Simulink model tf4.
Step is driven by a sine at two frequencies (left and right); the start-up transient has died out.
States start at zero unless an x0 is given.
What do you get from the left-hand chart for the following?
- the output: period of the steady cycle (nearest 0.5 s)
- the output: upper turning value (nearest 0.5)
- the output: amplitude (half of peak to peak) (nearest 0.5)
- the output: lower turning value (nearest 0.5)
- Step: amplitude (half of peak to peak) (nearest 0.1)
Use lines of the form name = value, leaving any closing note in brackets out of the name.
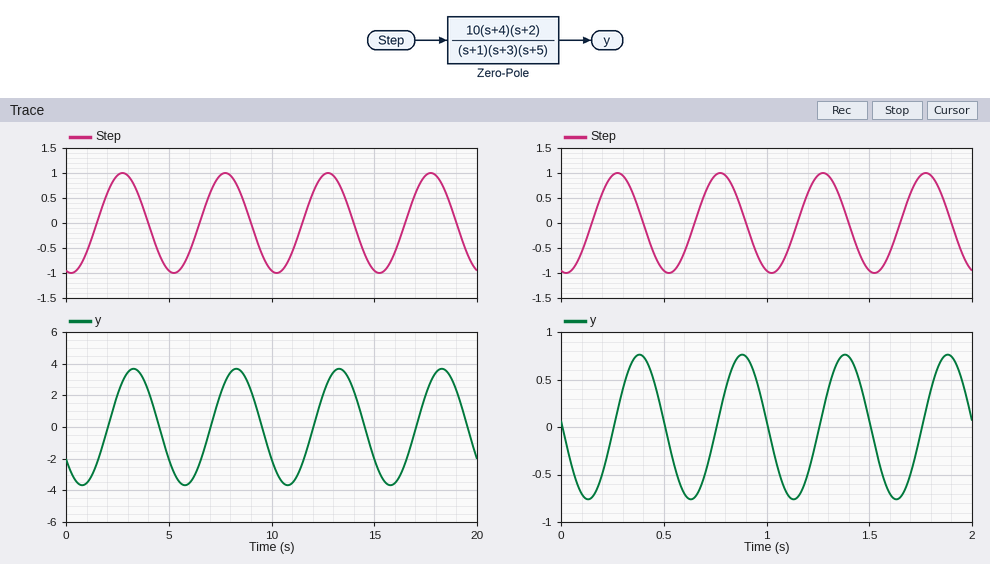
the output: period of the steady cycle = 5.0 s
the output: upper turning value = 3.5
the output: amplitude (half of peak to peak) = 3.5
the output: lower turning value = -3.5
Step: amplitude (half of peak to peak) = 1.0
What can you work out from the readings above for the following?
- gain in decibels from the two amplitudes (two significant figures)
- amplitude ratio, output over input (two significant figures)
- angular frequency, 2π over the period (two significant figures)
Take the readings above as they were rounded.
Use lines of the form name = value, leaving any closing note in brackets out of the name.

gain in decibels from the two amplitudes = 11 dB
amplitude ratio, output over input = 3.5
angular frequency, 2π over the period = 1.3 rad/s
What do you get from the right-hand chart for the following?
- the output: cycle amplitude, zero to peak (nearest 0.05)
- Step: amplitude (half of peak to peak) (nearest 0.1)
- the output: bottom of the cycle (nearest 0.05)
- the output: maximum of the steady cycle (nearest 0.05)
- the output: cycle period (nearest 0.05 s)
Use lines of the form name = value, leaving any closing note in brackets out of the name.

the output: cycle amplitude, zero to peak = 0.75
Step: amplitude (half of peak to peak) = 1.0
the output: bottom of the cycle = -0.75
the output: maximum of the steady cycle = 0.75
the output: cycle period = 0.50 s
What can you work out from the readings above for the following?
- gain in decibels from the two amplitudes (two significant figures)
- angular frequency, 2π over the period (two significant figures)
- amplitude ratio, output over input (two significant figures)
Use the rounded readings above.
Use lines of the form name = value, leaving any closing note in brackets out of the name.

gain in decibels from the two amplitudes = -2.5 dB
angular frequency, 2π over the period = 13 rad/s
amplitude ratio, output over input = 0.75
